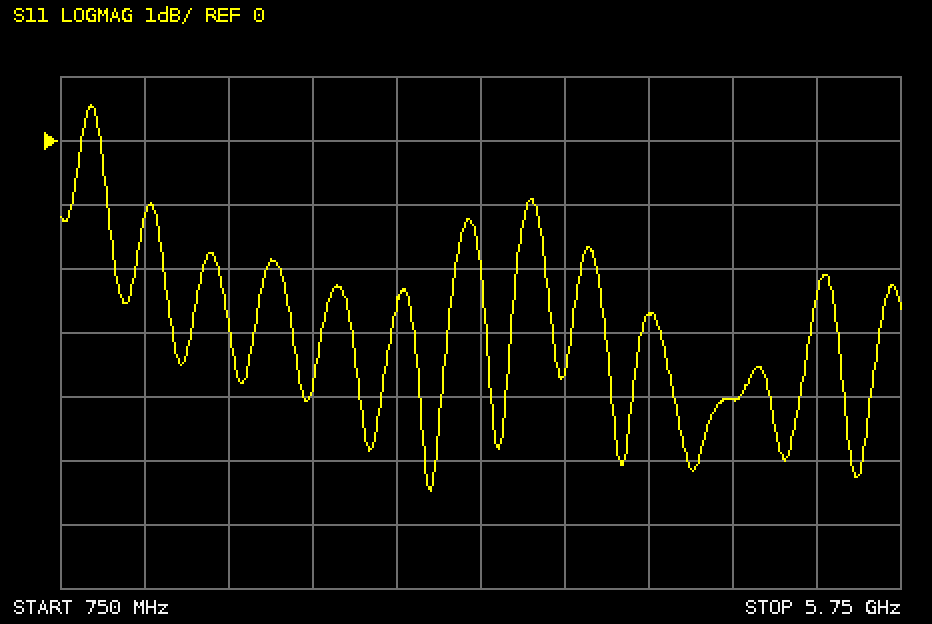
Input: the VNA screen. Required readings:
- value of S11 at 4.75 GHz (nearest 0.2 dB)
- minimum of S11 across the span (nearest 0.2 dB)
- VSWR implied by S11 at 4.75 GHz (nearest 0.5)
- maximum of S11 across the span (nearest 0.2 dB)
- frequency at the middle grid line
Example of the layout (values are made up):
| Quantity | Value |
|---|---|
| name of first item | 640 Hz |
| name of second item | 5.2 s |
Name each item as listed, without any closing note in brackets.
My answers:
| Quantity | Value |
|---|---|
| value of S11 at 4.75 GHz | -4.0 dB |
| minimum of S11 across the span | -5.4 dB |
| VSWR implied by S11 at 4.75 GHz | 4.5 |
| maximum of S11 across the span | 0.6 dB |
| frequency at the middle grid line | 3.25 GHz |
